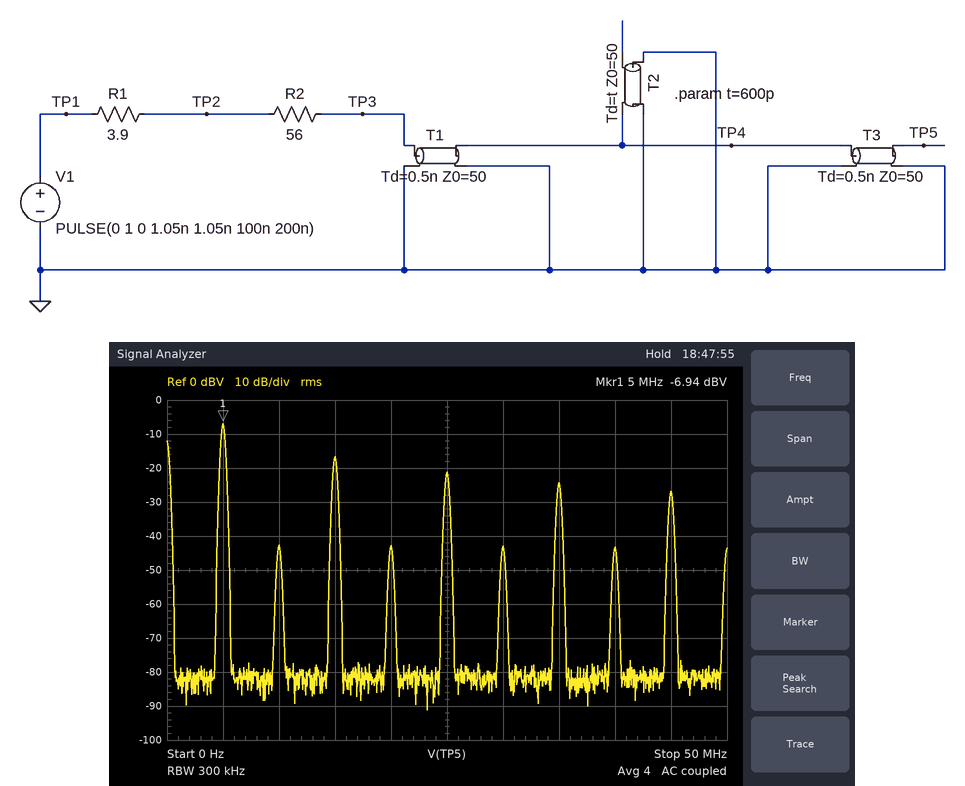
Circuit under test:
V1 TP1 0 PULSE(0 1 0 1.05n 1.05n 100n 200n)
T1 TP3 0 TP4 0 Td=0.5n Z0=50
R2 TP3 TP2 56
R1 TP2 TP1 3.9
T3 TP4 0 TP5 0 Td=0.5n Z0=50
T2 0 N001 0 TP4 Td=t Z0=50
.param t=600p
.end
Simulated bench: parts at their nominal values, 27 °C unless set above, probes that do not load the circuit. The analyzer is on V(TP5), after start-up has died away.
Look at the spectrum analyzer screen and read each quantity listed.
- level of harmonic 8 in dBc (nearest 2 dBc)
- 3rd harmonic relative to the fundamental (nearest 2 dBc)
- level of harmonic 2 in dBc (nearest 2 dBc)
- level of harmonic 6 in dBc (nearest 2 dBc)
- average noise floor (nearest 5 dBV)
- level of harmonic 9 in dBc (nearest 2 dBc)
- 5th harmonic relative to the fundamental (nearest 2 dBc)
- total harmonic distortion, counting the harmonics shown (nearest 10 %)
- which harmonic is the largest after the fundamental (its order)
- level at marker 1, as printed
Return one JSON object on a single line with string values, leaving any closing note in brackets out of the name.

{"level of harmonic 8 in dBc": "-36 dBc", "3rd harmonic relative to the fundamental": "-10 dBc", "level of harmonic 2 in dBc": "-36 dBc", "level of harmonic 6 in dBc": "-36 dBc", "average noise floor": "-80 dBV", "level of harmonic 9 in dBc": "-20 dBc", "5th harmonic relative to the fundamental": "-14 dBc", "total harmonic distortion, counting the harmonics shown": "40 %", "which harmonic is the largest after the fundamental": "3", "level at marker 1, as printed": "-6.94 dBV"}
